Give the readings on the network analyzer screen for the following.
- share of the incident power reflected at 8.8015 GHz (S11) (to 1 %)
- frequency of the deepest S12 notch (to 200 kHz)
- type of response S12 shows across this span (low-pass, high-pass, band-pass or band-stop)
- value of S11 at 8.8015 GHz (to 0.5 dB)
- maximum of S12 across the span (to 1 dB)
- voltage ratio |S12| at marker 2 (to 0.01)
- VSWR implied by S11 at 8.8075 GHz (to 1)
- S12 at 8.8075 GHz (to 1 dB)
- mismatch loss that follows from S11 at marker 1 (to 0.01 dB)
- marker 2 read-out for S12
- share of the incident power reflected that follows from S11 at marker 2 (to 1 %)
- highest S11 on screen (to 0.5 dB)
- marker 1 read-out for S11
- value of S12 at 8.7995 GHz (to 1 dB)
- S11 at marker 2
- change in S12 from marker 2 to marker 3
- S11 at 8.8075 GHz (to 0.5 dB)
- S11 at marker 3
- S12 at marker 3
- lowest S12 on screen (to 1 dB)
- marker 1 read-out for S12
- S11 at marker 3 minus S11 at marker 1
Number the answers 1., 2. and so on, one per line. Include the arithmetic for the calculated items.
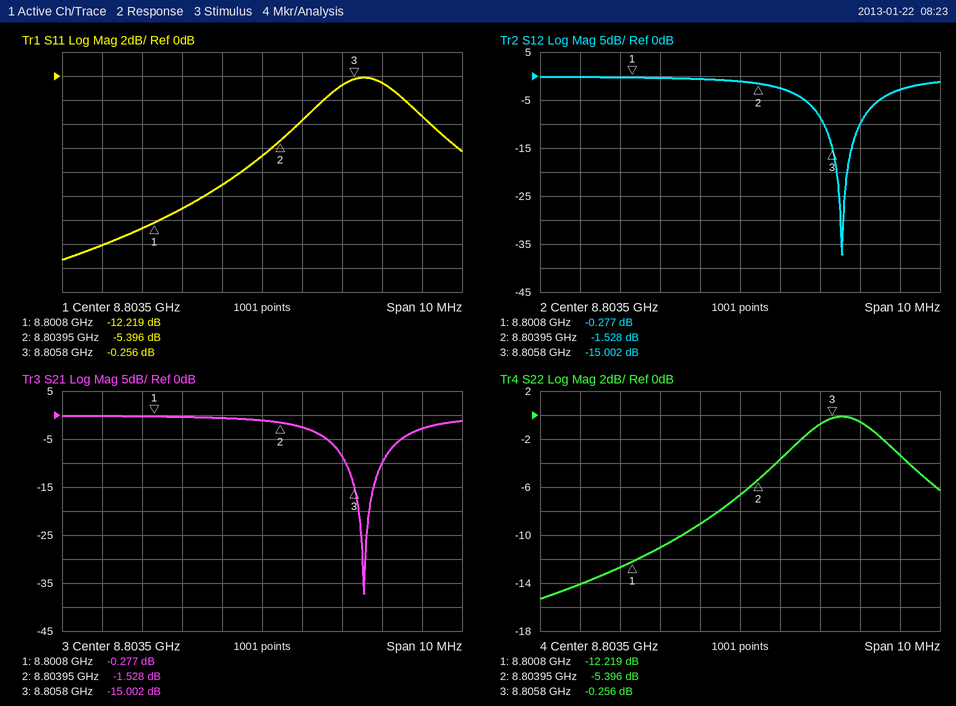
1. 10^(-11/10) ≈ 8 %
2. 8.8060 GHz
3. band-stop
4. -11.0 dB
5. 0 dB
6. 10^(-1.528/20) ≈ 0.84
7. |Γ| = 10^(-3.5/20) = 0.6683; VSWR = (1 + 0.6683)/(1 − 0.6683) ≈ 5
8. -3 dB
9. −10 log10(1 − 10^(-12.219/10)) ≈ 0.27 dB
10. -1.528 dB
11. 10^(-5.396/10) ≈ 29 %
12. 0.0 dB
13. -12.219 dB
14. 0 dB
15. -5.396 dB
16. -15.002 − (-1.528) = -13.474 dB
17. -3.5 dB
18. -0.256 dB
19. -15.002 dB
20. -37 dB
21. -0.277 dB
22. -0.256 − (-12.219) = 11.963 dB
